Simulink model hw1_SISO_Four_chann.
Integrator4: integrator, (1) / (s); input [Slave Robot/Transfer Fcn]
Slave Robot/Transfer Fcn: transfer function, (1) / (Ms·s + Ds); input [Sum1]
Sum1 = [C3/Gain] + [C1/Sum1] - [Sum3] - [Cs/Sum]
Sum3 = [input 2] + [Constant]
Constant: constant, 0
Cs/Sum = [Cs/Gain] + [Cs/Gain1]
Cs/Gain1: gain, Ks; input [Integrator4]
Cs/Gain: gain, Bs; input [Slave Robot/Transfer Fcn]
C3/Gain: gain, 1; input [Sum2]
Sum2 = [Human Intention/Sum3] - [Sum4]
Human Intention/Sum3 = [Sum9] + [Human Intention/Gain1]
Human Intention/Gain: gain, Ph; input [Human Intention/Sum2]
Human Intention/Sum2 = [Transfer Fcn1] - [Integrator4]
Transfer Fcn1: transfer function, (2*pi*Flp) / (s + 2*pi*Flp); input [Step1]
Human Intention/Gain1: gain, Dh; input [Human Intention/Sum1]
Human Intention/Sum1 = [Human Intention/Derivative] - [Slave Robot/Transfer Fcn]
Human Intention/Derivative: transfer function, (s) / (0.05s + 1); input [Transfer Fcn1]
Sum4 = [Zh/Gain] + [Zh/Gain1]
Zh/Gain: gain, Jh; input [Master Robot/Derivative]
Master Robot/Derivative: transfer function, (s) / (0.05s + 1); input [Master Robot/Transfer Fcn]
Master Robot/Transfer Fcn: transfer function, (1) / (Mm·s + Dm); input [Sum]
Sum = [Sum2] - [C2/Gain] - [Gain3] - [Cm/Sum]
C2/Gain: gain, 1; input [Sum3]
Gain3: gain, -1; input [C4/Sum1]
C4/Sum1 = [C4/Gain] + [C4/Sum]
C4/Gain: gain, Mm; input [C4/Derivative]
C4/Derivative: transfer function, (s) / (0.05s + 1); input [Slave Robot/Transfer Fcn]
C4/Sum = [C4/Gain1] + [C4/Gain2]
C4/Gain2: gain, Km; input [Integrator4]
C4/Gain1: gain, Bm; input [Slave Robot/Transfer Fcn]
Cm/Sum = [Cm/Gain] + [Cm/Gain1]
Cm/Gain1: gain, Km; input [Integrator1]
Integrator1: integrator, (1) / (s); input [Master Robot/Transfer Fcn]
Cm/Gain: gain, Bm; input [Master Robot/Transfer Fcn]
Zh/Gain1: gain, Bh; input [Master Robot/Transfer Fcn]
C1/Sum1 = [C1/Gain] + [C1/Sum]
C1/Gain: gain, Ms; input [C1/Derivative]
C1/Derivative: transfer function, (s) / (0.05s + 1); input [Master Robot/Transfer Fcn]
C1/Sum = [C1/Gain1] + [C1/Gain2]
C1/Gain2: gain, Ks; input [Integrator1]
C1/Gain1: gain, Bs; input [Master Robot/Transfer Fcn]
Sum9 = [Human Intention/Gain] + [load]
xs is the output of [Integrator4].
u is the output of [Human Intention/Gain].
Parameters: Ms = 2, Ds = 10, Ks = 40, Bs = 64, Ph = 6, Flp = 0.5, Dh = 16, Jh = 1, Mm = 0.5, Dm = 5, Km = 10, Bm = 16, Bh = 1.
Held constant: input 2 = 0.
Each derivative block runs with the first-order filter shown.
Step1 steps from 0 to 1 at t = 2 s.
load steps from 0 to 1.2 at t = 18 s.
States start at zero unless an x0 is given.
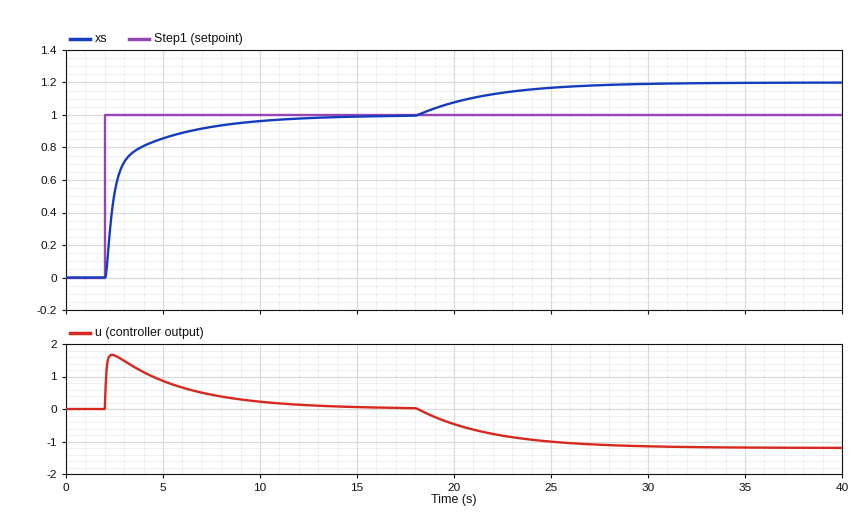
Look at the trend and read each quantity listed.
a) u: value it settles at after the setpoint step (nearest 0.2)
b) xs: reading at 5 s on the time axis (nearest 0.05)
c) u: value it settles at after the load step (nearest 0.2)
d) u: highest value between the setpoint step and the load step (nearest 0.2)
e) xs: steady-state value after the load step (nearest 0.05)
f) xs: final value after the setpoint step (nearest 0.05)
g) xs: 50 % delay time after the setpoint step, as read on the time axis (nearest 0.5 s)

0.0
0.85
-1.2
1.6
1.20
1.00
2.5 s
